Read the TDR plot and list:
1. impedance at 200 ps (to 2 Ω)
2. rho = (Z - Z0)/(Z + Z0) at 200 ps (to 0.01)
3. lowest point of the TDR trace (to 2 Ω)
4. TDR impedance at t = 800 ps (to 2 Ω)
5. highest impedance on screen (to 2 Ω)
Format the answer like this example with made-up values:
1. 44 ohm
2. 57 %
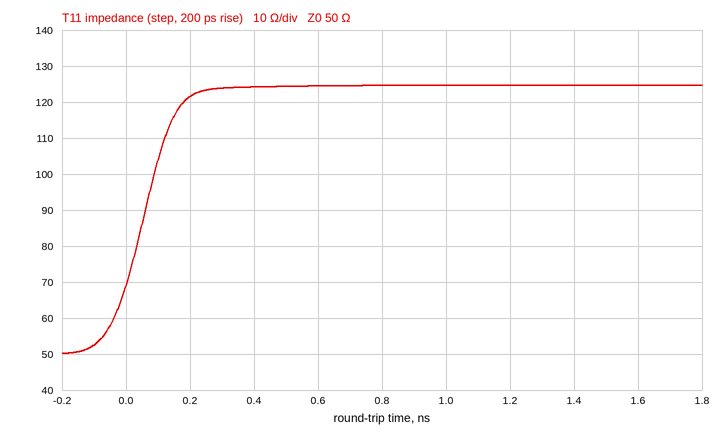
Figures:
1. 122 Ω
2. +0.42
3. 50 Ω
4. 124 Ω
5. 124 Ω
